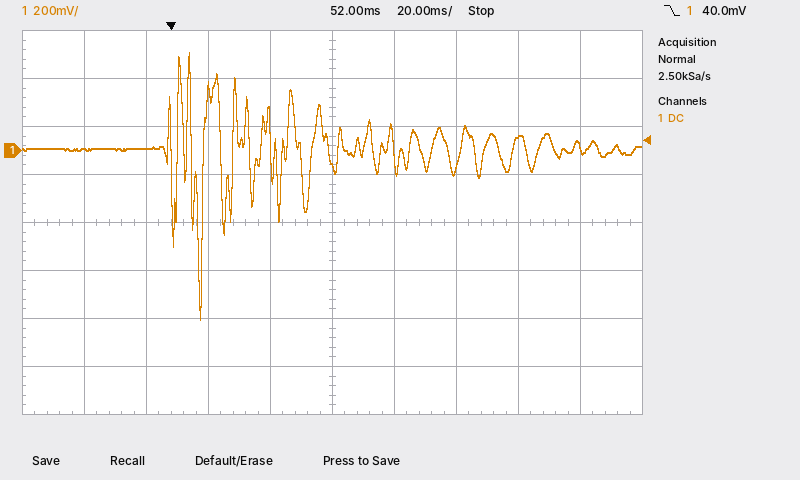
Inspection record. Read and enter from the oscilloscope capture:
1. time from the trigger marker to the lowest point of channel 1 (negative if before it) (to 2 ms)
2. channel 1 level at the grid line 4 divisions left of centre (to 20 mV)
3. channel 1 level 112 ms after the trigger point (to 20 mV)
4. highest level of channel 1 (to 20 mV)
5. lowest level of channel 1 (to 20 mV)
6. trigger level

+10 ms
0 mV
60 mV
400 mV
-700 mV
40.0 mV
